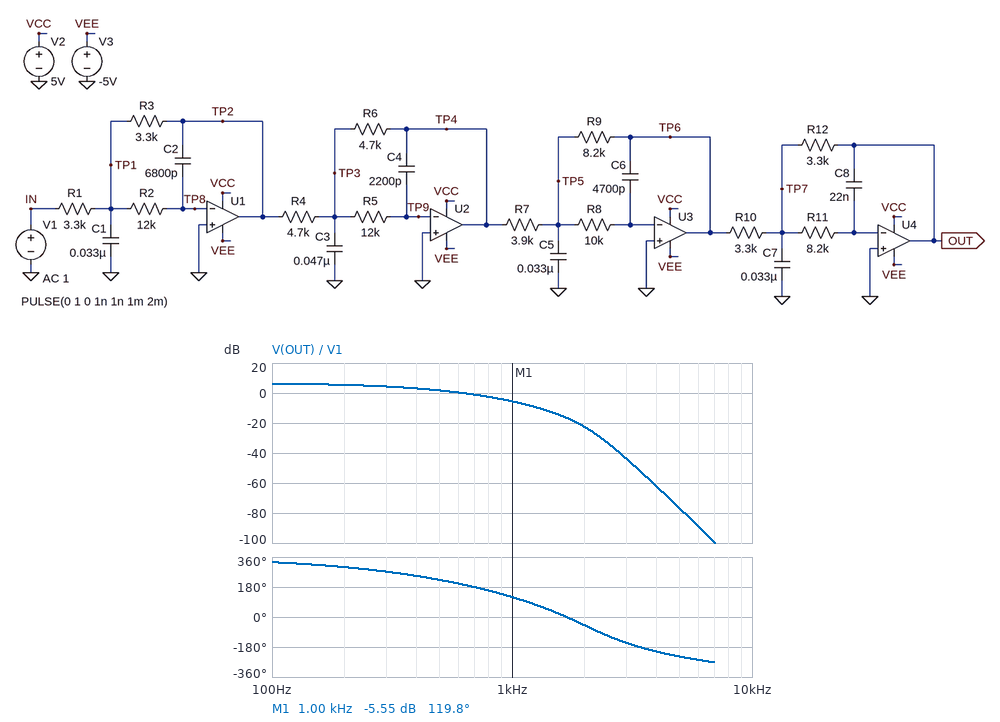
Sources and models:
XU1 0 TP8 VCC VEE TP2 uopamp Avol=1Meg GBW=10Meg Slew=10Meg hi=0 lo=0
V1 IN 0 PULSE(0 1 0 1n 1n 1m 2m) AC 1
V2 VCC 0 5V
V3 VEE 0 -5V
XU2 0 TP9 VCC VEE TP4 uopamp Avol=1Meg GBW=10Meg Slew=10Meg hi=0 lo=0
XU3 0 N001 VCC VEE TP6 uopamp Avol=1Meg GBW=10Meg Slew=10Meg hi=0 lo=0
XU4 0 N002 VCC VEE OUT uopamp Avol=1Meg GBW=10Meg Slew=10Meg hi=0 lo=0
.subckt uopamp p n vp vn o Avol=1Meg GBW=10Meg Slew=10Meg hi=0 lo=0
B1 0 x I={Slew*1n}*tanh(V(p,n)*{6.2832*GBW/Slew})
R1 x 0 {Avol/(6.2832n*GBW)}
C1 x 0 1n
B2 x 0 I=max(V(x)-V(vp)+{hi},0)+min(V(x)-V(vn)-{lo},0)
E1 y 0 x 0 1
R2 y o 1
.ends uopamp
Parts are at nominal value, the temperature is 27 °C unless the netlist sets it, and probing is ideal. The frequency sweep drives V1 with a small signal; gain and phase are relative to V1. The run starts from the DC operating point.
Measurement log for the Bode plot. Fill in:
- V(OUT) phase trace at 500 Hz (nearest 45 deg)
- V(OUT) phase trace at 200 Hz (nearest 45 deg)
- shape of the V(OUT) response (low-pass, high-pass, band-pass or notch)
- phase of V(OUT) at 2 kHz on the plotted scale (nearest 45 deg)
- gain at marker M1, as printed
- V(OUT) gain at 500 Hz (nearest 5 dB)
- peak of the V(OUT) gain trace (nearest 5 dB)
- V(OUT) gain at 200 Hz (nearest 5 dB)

225 deg
315 deg
low-pass
-45 deg
-5.55 dB
0 dB
5 dB
5 dB
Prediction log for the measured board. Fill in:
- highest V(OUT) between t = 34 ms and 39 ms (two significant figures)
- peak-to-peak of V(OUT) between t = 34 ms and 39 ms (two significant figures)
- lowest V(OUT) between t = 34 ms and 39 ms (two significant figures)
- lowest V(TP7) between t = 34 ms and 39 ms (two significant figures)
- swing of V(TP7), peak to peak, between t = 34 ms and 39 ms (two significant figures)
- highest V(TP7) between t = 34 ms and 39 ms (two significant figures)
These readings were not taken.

1.8 V
1.6 V
270 mV
-480 mV
960 mV
480 mV
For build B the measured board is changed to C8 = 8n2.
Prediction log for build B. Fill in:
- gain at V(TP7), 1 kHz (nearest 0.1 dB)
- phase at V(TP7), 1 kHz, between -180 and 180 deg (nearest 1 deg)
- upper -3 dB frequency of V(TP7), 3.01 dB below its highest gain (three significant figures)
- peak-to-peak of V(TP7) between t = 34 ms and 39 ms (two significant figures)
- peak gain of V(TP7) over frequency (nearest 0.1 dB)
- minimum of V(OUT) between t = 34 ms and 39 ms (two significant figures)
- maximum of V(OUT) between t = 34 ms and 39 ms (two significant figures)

-6.2 dB
60 deg
1.53 kHz
650 mV
-6.1 dB
2.3 mV
2.1 V
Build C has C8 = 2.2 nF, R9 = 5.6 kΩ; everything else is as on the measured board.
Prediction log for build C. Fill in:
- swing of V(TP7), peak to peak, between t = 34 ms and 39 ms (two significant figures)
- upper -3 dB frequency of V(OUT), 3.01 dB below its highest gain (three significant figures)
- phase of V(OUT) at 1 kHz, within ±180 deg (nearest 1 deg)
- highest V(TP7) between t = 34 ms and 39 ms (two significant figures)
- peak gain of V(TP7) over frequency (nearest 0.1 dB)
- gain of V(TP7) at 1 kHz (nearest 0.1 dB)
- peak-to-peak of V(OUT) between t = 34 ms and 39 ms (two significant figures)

180 mV
1.27 kHz
-158 deg
88 mV
-16.6 dB
-17.5 dB
1.5 V
